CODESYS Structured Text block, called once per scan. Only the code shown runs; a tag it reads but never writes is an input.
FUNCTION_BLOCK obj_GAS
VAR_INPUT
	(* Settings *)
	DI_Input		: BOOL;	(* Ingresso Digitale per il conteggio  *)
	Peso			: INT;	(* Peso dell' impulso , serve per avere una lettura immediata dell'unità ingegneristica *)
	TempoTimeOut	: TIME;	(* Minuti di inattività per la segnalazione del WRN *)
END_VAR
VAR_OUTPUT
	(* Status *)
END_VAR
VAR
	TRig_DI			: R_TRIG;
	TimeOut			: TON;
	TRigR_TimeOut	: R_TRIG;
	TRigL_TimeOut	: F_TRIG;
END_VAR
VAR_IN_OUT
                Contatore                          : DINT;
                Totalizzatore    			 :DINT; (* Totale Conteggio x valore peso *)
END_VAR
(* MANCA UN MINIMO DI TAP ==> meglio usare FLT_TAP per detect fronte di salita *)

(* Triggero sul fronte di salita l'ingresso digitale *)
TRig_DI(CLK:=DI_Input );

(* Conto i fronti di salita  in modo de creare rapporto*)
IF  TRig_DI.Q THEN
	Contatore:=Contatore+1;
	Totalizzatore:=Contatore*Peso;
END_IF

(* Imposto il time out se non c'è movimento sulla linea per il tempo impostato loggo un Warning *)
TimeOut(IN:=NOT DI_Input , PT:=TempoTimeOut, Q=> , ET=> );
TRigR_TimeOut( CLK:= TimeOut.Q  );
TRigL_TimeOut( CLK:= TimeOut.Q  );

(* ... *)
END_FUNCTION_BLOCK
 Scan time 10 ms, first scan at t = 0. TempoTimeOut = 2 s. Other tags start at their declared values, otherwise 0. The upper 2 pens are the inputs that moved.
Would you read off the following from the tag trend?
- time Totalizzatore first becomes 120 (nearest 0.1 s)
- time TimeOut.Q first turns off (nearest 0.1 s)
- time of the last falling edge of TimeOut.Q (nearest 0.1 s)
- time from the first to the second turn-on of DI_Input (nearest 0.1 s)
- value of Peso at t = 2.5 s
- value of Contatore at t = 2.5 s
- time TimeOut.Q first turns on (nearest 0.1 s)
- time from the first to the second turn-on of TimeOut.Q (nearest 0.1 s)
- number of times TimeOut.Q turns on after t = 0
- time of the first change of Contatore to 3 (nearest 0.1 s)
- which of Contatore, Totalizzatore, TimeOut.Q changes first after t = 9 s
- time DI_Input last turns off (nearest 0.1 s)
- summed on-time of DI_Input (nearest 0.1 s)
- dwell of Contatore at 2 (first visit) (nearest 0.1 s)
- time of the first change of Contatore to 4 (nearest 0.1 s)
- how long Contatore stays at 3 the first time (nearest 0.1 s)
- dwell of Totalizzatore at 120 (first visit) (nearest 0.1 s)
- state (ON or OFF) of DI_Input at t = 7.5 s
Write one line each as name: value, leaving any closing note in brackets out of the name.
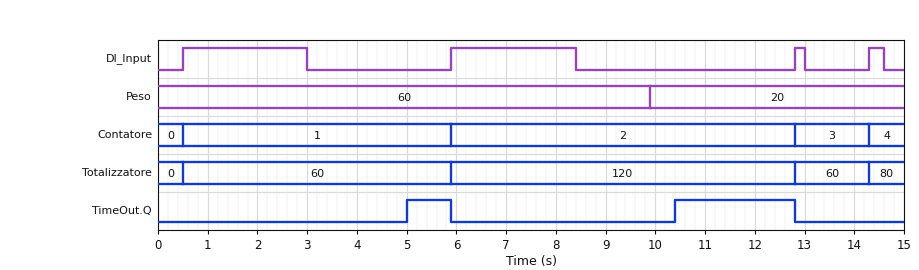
time Totalizzatore first becomes 120: 5.9 s
time TimeOut.Q first turns off: 5.9 s
time of the last falling edge of TimeOut.Q: 12.8 s
time from the first to the second turn-on of DI_Input: 5.4 s
value of Peso at t = 2.5 s: 60
value of Contatore at t = 2.5 s: 1
time TimeOut.Q first turns on: 5.0 s
time from the first to the second turn-on of TimeOut.Q: 5.4 s
number of times TimeOut.Q turns on after t = 0: 2
time of the first change of Contatore to 3: 12.8 s
which of Contatore, Totalizzatore, TimeOut.Q changes first after t = 9 s: TimeOut.Q
time DI_Input last turns off: 14.6 s
summed on-time of DI_Input: 5.5 s
dwell of Contatore at 2 (first visit): 6.9 s
time of the first change of Contatore to 4: 14.3 s
how long Contatore stays at 3 the first time: 1.5 s
dwell of Totalizzatore at 120 (first visit): 6.9 s
state (ON or OFF) of DI_Input at t = 7.5 s: ON
